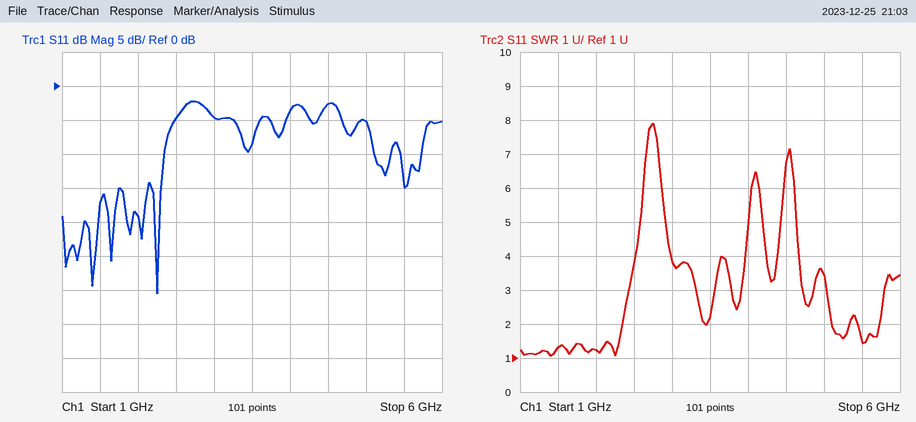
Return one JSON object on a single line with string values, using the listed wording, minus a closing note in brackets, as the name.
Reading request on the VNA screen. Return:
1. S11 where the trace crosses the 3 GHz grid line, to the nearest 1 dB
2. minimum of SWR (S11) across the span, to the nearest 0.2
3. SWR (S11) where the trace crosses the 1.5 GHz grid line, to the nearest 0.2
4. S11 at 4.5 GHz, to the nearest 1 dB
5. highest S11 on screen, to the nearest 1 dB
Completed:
{"S11 where the trace crosses the 3 GHz grid line, to the nearest 1 dB": "-5 dB", "minimum of SWR (S11) across the span, to the nearest 0.2": "1.0", "SWR (S11) where the trace crosses the 1.5 GHz grid line, to the nearest 0.2": "1.4", "S11 at 4.5 GHz, to the nearest 1 dB": "-3 dB", "highest S11 on screen, to the nearest 1 dB": "-2 dB"}
